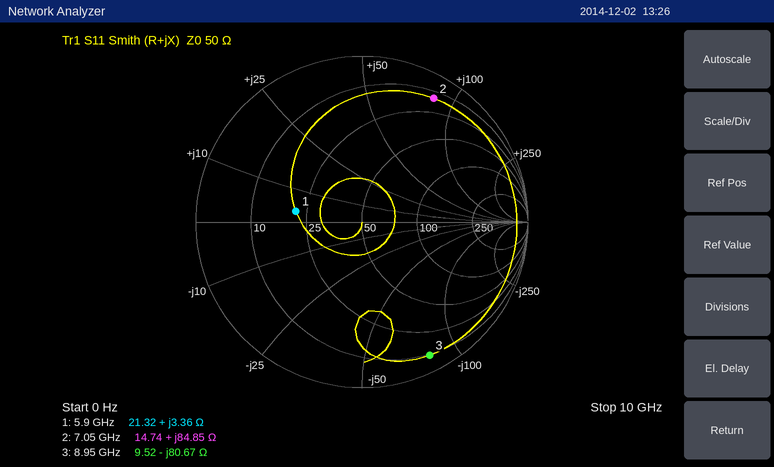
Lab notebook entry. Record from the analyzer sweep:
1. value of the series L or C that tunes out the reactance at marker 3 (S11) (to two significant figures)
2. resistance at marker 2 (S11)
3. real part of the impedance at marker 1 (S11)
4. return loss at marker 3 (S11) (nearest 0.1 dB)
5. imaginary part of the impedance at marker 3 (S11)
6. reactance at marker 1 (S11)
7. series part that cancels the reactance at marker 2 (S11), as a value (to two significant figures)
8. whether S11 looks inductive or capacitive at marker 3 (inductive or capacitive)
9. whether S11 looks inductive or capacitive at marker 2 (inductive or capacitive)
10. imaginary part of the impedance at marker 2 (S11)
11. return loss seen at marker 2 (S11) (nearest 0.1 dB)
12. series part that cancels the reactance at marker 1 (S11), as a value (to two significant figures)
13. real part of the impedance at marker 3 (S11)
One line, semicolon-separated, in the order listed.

1.4 nH; 14.74 Ω; 21.32 Ω; 0.9 dB; -80.67 Ω; +3.36 Ω; 270 fF; capacitive; inductive; +84.85 Ω; 1.3 dB; 8.0 pF; 9.52 Ω
